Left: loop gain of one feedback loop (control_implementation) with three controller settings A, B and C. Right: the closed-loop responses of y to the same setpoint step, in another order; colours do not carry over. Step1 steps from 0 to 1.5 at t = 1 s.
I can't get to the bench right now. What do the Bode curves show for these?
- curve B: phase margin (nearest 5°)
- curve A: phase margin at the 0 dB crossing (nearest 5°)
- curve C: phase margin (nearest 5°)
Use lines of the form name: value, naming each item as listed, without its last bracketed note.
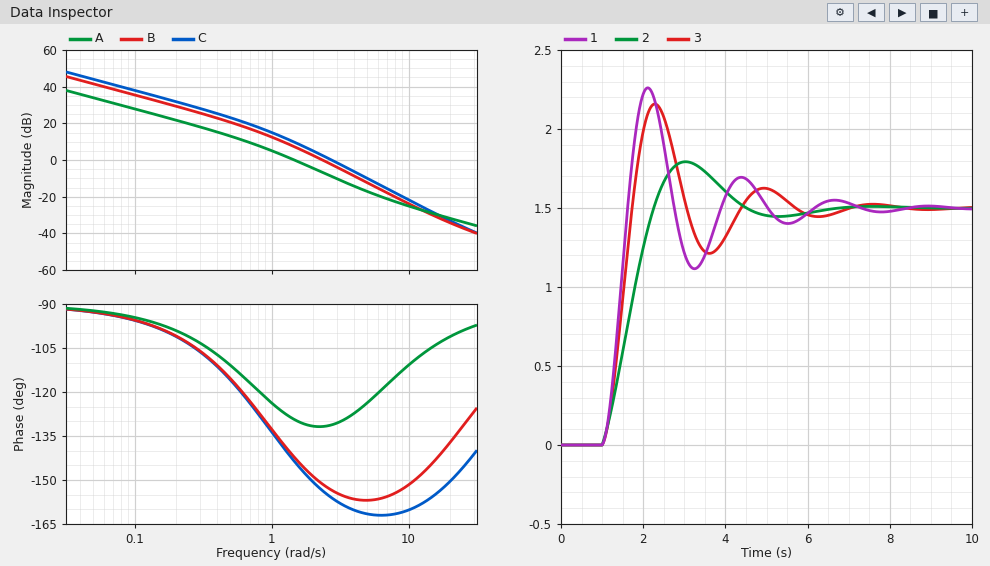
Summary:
curve B: phase margin: 30°
curve A: phase margin at the 0 dB crossing: 50°
curve C: phase margin: 25°
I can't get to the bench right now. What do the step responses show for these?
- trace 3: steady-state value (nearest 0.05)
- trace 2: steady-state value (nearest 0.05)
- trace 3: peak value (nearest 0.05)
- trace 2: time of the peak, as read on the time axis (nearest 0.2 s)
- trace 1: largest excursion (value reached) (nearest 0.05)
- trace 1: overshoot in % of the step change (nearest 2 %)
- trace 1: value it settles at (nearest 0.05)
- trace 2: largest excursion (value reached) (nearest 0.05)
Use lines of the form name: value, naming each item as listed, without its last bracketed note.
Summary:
trace 3: steady-state value: 1.50
trace 2: steady-state value: 1.50
trace 3: peak value: 2.15
trace 2: time of the peak, as read on the time axis: 3.0 s
trace 1: largest excursion (value reached): 2.25
trace 1: overshoot in % of the step change: 50 %
trace 1: value it settles at: 1.50
trace 2: largest excursion (value reached): 1.80
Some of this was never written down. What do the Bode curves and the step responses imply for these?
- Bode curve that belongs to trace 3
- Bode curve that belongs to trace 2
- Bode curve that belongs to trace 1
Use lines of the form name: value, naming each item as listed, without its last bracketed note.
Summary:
Bode curve that belongs to trace 3: B
Bode curve that belongs to trace 2: A
Bode curve that belongs to trace 1: C
